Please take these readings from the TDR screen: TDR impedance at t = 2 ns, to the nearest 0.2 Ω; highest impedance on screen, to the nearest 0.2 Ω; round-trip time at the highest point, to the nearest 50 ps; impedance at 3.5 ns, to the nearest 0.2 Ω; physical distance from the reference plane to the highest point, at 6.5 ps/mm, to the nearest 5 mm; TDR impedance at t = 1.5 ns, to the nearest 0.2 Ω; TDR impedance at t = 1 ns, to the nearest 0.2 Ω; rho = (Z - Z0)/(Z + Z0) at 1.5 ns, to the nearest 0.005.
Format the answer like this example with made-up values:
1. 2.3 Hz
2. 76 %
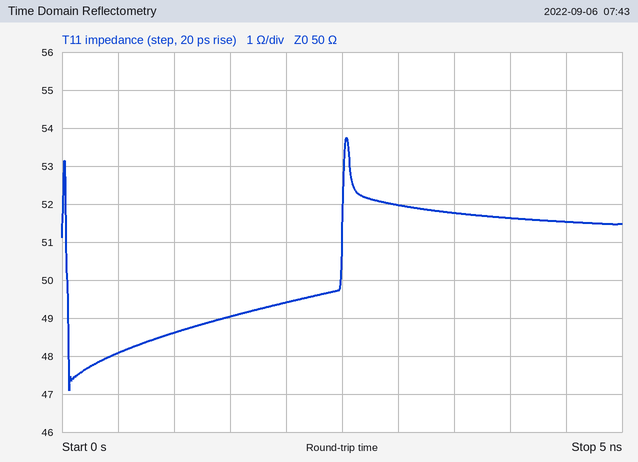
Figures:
1. 49.4 Ω
2. 53.8 Ω
3. 2.55 ns
4. 51.8 Ω
5. 195 mm
6. 49.0 Ω
7. 48.6 Ω
8. -0.010
